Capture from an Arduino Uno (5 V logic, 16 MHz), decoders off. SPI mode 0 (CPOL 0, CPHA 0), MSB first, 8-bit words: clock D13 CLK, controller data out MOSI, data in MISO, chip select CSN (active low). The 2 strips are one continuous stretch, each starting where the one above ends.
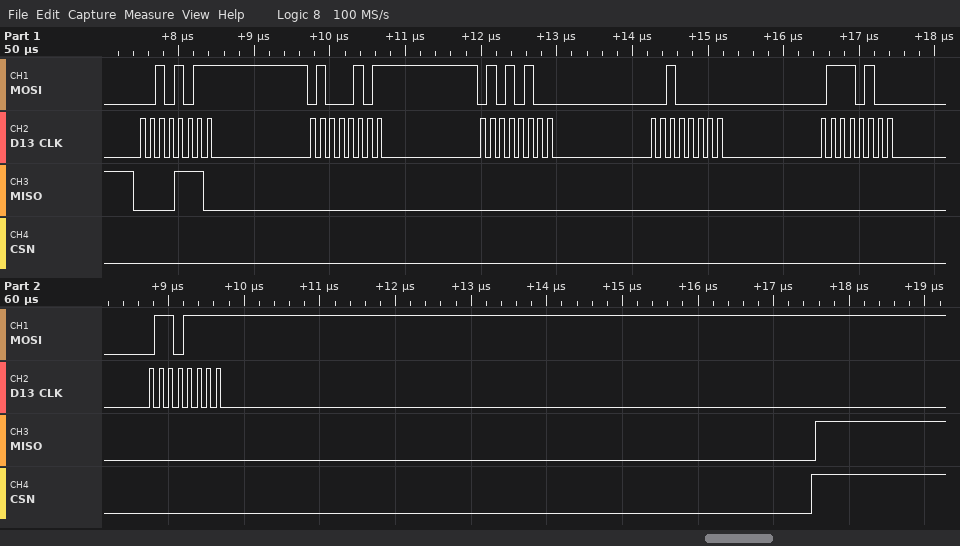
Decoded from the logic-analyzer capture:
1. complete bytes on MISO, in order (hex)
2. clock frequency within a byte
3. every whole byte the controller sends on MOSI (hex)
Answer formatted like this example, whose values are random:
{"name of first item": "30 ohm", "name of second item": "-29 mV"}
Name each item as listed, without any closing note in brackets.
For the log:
{"complete bytes on MISO, in order": "0x0E 0x00 0x00 0x00 0x00 0x00", "clock frequency within a byte": "8 MHz", "every whole byte the controller sends on MOSI": "0x2B 0x45 0x54 0x20 0x74 0x6F"}
